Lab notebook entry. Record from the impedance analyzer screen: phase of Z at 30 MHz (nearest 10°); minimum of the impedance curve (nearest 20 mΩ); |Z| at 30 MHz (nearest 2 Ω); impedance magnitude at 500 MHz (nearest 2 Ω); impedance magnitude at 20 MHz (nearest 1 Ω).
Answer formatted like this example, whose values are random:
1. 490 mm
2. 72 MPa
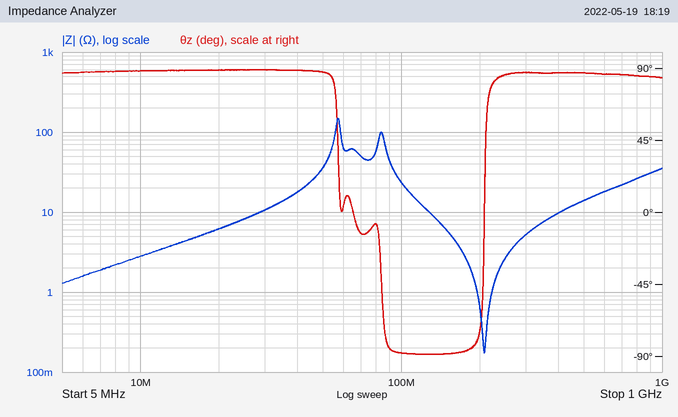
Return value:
1. 90°
2. 180 mΩ
3. 10 Ω
4. 14 Ω
5. 6 Ω
